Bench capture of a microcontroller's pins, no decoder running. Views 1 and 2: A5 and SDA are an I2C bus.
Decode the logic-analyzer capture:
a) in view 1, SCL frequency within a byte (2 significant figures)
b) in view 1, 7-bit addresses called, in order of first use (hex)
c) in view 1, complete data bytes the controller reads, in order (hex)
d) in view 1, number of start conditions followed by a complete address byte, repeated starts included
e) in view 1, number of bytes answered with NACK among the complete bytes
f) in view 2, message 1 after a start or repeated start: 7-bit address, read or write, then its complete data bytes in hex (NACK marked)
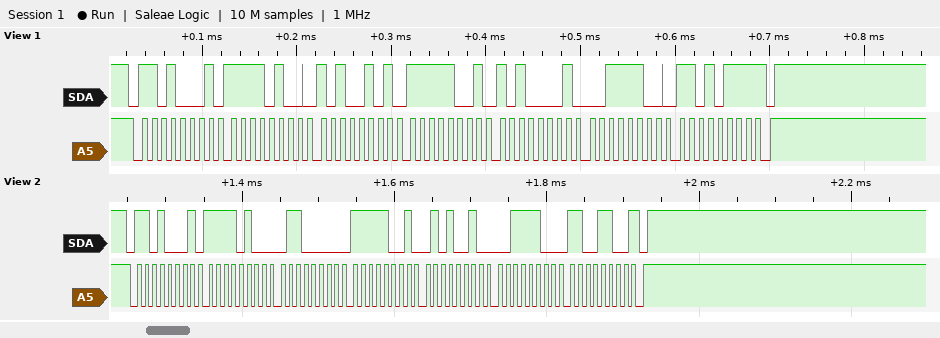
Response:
100 kHz
0x68
F4 A5 F9 A1 3C D7
1
1
0x68 read: F4 60 F9 52 3C CC NACK
